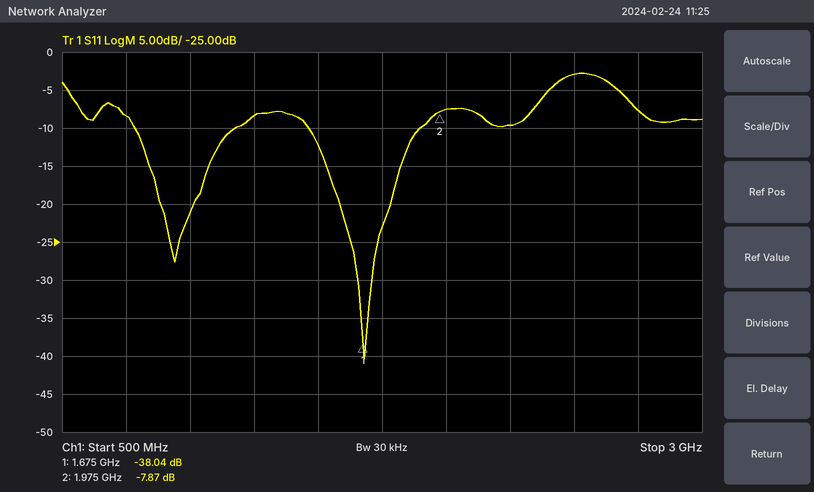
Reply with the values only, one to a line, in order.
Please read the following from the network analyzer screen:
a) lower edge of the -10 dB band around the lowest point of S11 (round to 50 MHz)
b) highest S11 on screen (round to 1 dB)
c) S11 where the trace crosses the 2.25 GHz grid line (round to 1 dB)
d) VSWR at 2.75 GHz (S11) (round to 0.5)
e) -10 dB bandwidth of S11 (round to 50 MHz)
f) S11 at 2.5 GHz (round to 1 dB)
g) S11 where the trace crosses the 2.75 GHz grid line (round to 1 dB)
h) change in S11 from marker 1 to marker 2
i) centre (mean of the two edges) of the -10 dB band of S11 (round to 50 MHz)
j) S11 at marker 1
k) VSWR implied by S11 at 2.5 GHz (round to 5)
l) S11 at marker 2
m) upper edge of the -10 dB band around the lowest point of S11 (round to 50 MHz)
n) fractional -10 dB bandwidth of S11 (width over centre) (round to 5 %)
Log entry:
1.45 GHz
-3 dB
-10 dB
2.5
450 MHz
-3 dB
-8 dB
30.17 dB
1.70 GHz
-38.04 dB
5
-7.87 dB
1.90 GHz
25 %
